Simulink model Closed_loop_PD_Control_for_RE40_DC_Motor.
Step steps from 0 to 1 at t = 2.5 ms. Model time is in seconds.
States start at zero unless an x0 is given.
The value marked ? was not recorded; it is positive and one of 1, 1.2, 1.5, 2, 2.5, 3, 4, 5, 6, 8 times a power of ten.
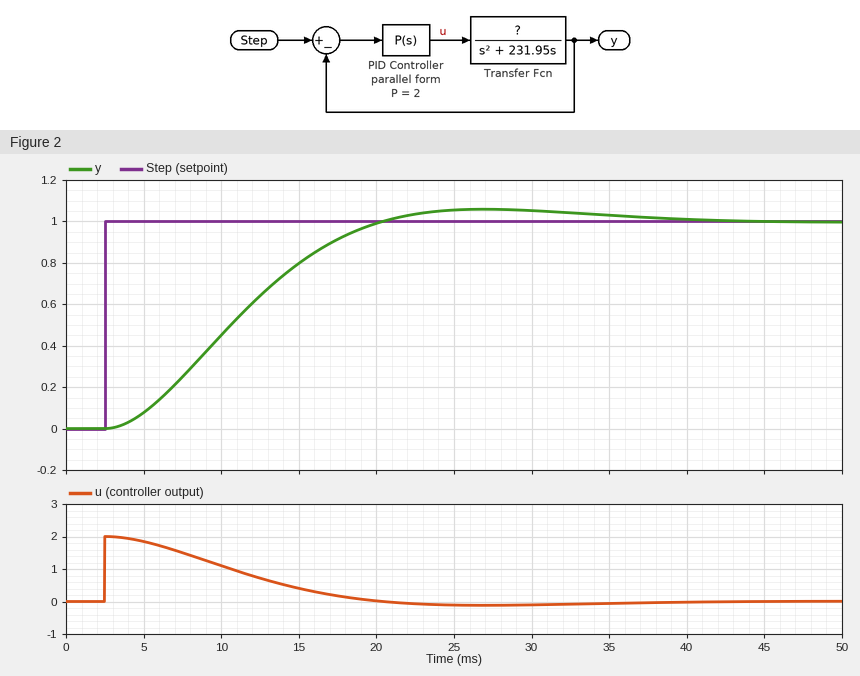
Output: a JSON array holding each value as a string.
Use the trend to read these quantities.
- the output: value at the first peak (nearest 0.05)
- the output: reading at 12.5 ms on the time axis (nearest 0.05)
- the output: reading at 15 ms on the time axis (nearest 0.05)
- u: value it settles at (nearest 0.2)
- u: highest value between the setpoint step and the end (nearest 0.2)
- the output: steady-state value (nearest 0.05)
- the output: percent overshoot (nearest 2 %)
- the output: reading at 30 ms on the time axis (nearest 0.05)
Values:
["1.05", "0.65", "0.80", "0.0", "2.0", "1.00", "6 %", "1.05"]
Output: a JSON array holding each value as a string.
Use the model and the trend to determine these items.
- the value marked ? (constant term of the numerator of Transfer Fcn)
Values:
["15000"]
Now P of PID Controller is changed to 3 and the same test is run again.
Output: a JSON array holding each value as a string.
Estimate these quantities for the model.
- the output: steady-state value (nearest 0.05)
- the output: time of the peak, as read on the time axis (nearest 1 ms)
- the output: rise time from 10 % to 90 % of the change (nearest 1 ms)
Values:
["1.00", "20 ms", "8 ms"]
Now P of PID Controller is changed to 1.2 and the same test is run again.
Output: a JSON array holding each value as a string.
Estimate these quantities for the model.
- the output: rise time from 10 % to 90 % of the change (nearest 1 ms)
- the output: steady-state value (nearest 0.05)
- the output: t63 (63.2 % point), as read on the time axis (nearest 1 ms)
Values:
["20 ms", "1.00", "17 ms"]
